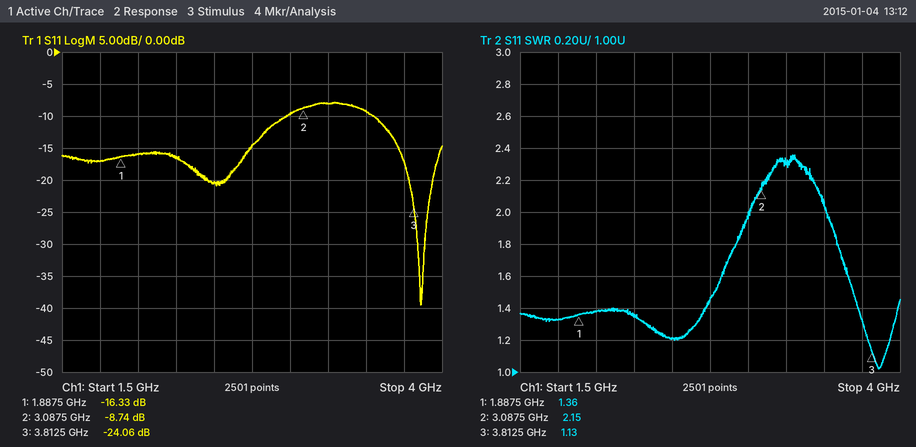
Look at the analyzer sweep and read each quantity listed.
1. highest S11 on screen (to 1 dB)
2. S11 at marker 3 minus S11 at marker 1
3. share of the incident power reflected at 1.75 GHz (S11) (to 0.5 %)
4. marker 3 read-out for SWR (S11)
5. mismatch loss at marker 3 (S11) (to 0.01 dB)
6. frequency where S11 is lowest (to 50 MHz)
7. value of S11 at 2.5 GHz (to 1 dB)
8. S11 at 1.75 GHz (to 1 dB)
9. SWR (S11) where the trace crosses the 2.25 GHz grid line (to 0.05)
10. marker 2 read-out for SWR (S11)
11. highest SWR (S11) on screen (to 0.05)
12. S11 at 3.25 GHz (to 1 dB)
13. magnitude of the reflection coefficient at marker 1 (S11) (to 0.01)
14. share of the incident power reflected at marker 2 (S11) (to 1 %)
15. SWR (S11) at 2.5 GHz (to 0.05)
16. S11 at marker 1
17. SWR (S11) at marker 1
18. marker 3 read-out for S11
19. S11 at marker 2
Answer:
-8 dB
-7.73 dB
2.0 %
1.13
0.02 dB
3.85 GHz
-20 dB
-17 dB
1.35
2.15
2.35
-8 dB
0.15
13 %
1.20
-16.33 dB
1.36
-24.06 dB
-8.74 dB
